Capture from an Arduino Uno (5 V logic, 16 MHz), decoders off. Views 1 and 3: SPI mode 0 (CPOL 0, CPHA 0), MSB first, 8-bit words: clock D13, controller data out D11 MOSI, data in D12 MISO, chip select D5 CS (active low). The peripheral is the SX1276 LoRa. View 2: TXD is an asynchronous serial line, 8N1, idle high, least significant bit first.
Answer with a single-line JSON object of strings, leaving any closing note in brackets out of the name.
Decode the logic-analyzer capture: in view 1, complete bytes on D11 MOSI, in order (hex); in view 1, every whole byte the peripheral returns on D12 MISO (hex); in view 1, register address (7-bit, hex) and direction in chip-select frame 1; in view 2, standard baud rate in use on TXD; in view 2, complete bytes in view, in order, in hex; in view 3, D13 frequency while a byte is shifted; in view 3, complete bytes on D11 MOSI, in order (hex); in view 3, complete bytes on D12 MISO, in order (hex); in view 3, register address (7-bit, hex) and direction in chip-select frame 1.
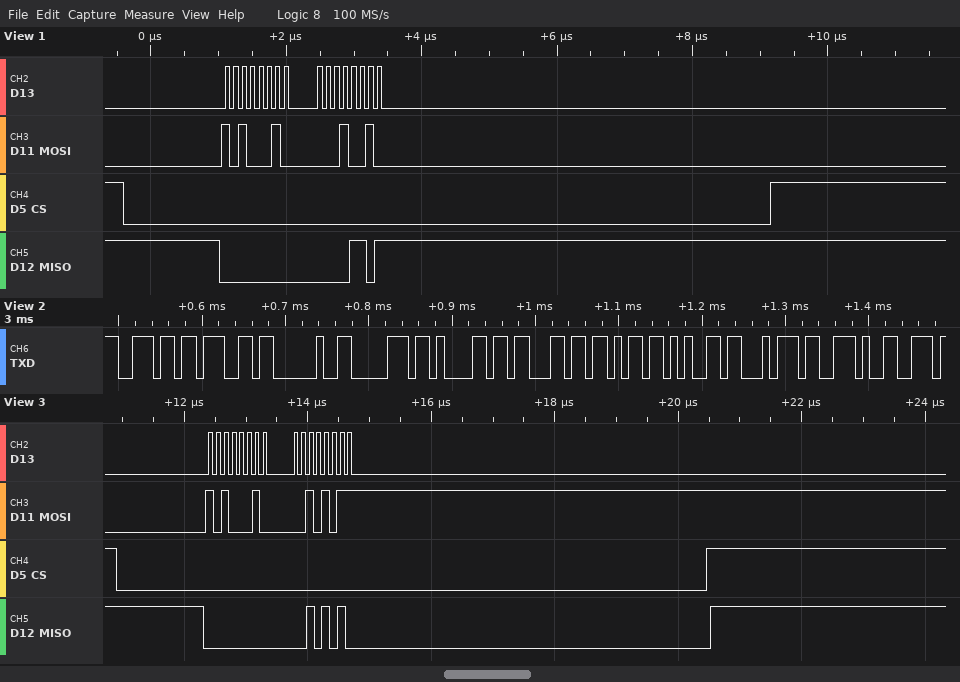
{"in view 1, complete bytes on D11 MOSI, in order": "0xA2 0x12", "in view 1, every whole byte the peripheral returns on D12 MISO": "0x00 0x0D", "in view 1, register address (7-bit, hex) and direction in chip-select frame 1": "0x22 write", "in view 2, standard baud rate in use on TXD": "115200 baud", "in view 2, complete bytes in view, in order, in hex": "0x6E 0x67 0x20 0x70 0x61 0x63 0x6B 0x65 0x74 0x2E", "in view 3, D13 frequency while a byte is shifted": "8 MHz", "in view 3, complete bytes on D11 MOSI, in order": "A2 2B", "in view 3, complete bytes on D12 MISO, in order": "00 2A", "in view 3, register address (7-bit, hex) and direction in chip-select frame 1": "0x22 write"}
